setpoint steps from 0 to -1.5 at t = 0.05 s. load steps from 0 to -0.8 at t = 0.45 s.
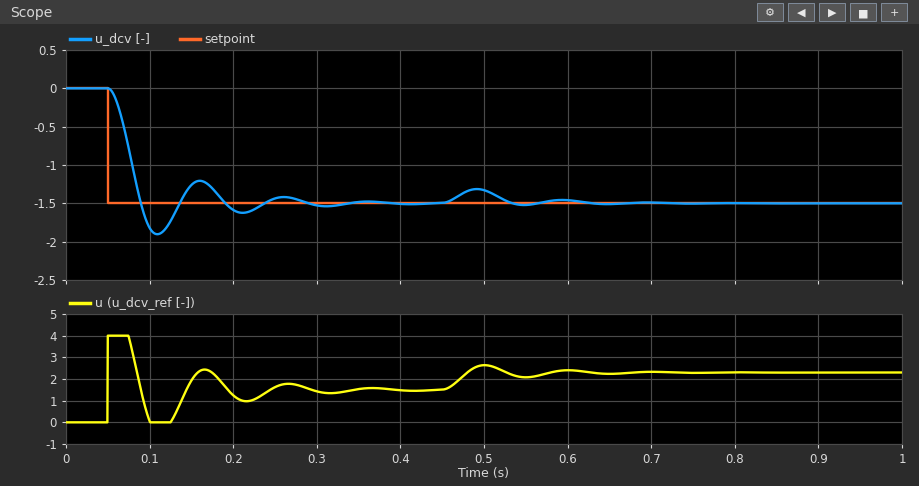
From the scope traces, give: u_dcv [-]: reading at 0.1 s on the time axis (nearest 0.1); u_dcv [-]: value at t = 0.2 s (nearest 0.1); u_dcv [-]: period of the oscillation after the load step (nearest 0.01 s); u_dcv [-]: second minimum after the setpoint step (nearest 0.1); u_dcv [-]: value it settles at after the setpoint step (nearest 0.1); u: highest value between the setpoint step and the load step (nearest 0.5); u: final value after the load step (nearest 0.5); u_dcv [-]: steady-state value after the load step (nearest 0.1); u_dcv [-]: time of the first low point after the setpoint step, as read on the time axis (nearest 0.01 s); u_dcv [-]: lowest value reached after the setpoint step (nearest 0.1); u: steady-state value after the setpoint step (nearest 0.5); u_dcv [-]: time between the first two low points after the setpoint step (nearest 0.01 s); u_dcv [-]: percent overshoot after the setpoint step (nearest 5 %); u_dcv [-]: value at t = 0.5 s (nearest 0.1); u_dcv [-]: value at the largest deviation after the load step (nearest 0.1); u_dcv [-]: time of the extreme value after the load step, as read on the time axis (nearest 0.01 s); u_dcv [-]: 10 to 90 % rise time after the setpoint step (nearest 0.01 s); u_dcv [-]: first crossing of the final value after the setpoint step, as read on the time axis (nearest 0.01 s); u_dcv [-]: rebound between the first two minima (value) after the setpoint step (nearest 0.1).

-1.8
-1.6
0.10 s
-1.6
-1.5
4.0
2.5
-1.5
0.11 s
-1.9
1.5
0.10 s
25 %
-1.3
-1.3
0.49 s
0.03 s
0.09 s
-1.2
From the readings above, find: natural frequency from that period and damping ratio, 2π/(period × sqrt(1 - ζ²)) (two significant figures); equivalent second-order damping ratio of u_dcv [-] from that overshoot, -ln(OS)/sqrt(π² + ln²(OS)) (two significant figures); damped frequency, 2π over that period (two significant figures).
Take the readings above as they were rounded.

69 rad/s
0.40
63 rad/s
